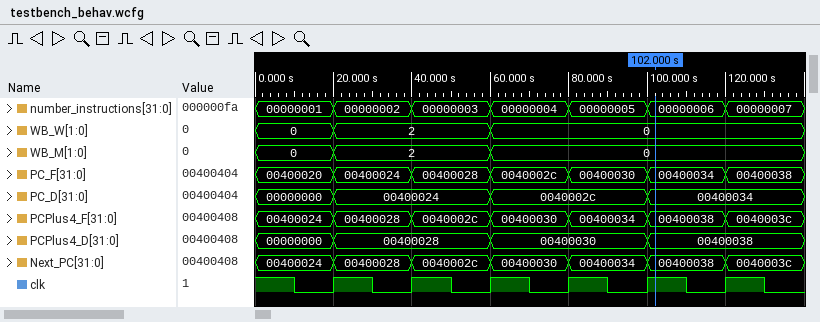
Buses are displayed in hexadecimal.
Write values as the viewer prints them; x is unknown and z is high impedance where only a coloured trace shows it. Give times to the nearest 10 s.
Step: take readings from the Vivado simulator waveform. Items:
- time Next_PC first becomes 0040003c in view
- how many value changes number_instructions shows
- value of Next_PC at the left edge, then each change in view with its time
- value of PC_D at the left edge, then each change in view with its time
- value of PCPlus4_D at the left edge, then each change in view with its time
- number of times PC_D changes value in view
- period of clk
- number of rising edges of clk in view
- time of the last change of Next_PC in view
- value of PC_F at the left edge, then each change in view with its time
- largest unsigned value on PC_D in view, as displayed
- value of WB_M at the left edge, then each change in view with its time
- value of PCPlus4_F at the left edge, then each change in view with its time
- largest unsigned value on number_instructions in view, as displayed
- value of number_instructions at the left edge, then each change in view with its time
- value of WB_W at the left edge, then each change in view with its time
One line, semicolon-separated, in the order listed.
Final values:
120 s; 6; 00400024, 00400028 at 20 s, 0040002c at 40 s, 00400030 at 60 s, 00400034 at 80 s, 00400038 at 100 s, 0040003c at 120 s; 00000000, 00400024 at 20 s, 0040002c at 60 s, 00400034 at 100 s; 00000000, 00400028 at 20 s, 00400030 at 60 s, 00400038 at 100 s; 3; 20 s; 6; 120 s; 00400020, 00400024 at 20 s, 00400028 at 40 s, 0040002c at 60 s, 00400030 at 80 s, 00400034 at 100 s, 00400038 at 120 s; 00400034; 0, 2 at 20 s, 0 at 60 s; 00400024, 00400028 at 20 s, 0040002c at 40 s, 00400030 at 60 s, 00400034 at 80 s, 00400038 at 100 s, 0040003c at 120 s; 00000007; 00000001, 00000002 at 20 s, 00000003 at 40 s, 00000004 at 60 s, 00000005 at 80 s, 00000006 at 100 s, 00000007 at 120 s; 0, 2 at 20 s, 0 at 60 s
